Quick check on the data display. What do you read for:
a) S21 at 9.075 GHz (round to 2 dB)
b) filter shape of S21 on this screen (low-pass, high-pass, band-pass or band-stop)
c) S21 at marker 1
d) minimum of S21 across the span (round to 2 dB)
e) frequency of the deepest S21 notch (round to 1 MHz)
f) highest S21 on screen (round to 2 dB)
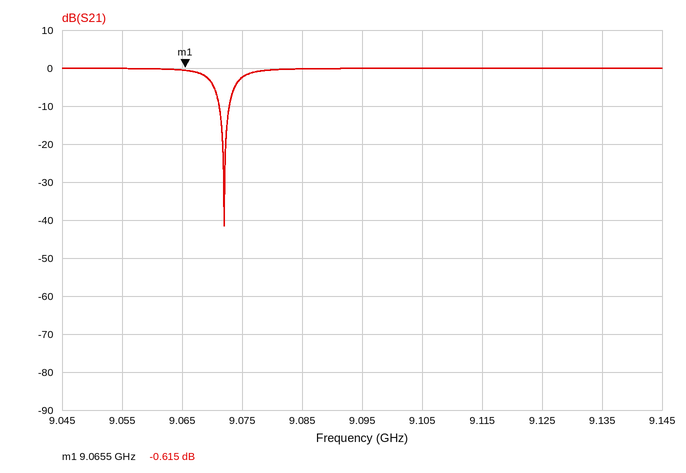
-2 dB
band-stop
-0.615 dB
-42 dB
9.072 GHz
0 dB
